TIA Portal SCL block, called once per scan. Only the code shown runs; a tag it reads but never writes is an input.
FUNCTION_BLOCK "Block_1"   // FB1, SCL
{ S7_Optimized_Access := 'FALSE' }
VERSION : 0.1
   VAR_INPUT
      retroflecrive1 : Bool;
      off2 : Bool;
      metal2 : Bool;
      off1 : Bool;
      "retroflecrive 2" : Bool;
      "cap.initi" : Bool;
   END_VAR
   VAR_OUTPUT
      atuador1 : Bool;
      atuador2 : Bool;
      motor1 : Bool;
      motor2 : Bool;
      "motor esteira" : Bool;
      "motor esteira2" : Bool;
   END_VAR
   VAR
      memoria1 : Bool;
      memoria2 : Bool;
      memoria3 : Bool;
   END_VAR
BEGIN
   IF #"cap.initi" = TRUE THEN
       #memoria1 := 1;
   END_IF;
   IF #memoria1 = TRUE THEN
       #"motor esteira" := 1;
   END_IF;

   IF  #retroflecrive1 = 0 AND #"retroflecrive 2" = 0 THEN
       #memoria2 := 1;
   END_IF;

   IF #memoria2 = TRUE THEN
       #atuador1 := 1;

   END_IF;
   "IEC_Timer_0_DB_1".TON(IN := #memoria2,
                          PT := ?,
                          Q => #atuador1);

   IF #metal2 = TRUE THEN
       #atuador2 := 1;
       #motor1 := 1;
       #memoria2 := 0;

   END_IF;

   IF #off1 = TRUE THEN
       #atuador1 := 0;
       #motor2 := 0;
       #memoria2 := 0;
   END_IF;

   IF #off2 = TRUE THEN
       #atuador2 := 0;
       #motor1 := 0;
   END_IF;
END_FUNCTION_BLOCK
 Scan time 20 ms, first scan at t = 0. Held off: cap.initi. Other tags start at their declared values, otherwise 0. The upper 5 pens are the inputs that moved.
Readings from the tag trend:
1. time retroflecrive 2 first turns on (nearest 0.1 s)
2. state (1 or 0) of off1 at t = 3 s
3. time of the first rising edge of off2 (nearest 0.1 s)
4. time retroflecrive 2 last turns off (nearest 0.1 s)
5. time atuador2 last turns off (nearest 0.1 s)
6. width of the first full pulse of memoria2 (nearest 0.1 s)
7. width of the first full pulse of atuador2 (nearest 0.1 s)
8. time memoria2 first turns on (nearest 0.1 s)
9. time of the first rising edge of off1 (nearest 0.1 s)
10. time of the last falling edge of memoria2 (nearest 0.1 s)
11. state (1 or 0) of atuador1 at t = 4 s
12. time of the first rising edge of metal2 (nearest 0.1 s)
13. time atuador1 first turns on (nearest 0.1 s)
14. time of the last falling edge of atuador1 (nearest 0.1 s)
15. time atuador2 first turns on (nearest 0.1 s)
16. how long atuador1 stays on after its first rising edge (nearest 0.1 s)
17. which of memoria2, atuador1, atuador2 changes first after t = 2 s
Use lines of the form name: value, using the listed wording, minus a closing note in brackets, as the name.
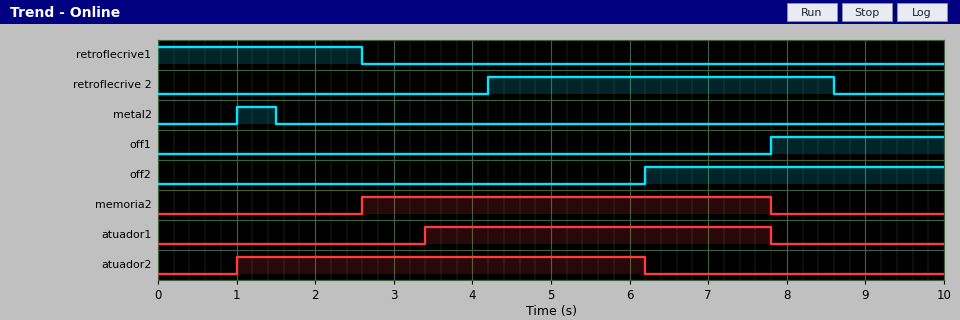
time retroflecrive 2 first turns on: 4.2 s
state (1 or 0) of off1 at t = 3 s: 0
time of the first rising edge of off2: 6.2 s
time retroflecrive 2 last turns off: 8.6 s
time atuador2 last turns off: 6.2 s
width of the first full pulse of memoria2: 5.2 s
width of the first full pulse of atuador2: 5.2 s
time memoria2 first turns on: 2.6 s
time of the first rising edge of off1: 7.8 s
time of the last falling edge of memoria2: 7.8 s
state (1 or 0) of atuador1 at t = 4 s: 1
time of the first rising edge of metal2: 1.0 s
time atuador1 first turns on: 3.4 s
time of the last falling edge of atuador1: 7.8 s
time atuador2 first turns on: 1.0 s
how long atuador1 stays on after its first rising edge: 4.4 s
which of memoria2, atuador1, atuador2 changes first after t = 2 s: memoria2
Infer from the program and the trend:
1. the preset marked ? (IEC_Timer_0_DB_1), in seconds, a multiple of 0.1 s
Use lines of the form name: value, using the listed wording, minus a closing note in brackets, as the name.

the preset marked ? (IEC_Timer_0_DB_1), in seconds, a multiple of 0.1 s: 0.8 s
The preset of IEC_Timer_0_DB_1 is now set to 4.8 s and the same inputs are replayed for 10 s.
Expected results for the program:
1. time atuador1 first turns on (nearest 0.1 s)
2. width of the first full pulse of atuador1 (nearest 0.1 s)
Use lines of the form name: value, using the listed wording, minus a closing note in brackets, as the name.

time atuador1 first turns on: 7.4 s
width of the first full pulse of atuador1: 0.4 s
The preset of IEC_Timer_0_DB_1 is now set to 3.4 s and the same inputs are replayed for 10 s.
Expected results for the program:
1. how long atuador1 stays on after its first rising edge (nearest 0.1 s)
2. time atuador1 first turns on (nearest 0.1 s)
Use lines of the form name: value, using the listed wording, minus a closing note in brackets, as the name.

how long atuador1 stays on after its first rising edge: 1.8 s
time atuador1 first turns on: 6.0 s
